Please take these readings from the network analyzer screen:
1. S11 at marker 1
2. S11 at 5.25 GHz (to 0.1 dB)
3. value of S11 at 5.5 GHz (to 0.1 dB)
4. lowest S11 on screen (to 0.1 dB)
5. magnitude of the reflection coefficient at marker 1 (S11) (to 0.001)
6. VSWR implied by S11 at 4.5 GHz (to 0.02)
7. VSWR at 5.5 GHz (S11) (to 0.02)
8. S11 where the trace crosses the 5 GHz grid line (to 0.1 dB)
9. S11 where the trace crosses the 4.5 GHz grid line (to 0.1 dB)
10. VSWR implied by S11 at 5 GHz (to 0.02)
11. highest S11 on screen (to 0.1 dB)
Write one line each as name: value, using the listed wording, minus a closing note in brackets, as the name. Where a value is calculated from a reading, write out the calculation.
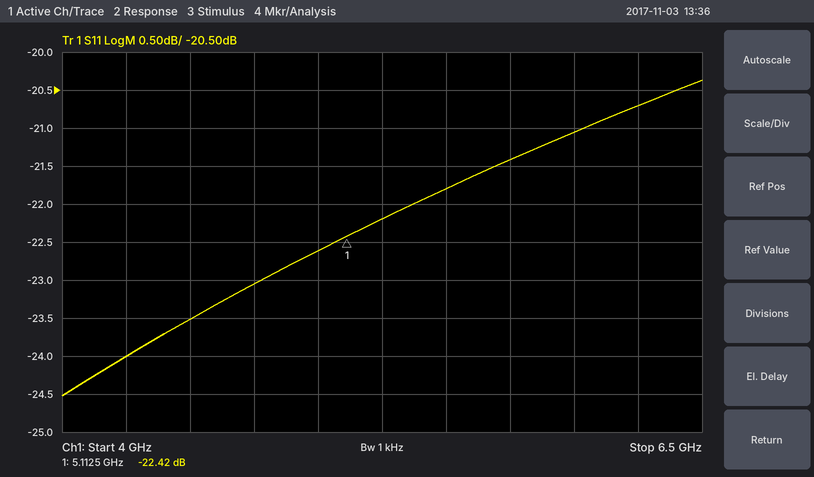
S11 at marker 1: -22.42 dB
S11 at 5.25 GHz: -22.2 dB
value of S11 at 5.5 GHz: -21.8 dB
lowest S11 on screen: -24.5 dB
magnitude of the reflection coefficient at marker 1 (S11): 10^(-22.42/20) ≈ 0.076
VSWR implied by S11 at 4.5 GHz: |Γ| = 10^(-23.5/20) = 0.0668; VSWR = (1 + 0.0668)/(1 − 0.0668) ≈ 1.14
VSWR at 5.5 GHz (S11): |Γ| = 10^(-21.8/20) = 0.0813; VSWR = (1 + 0.0813)/(1 − 0.0813) ≈ 1.18
S11 where the trace crosses the 5 GHz grid line: -22.6 dB
S11 where the trace crosses the 4.5 GHz grid line: -23.5 dB
VSWR implied by S11 at 5 GHz: |Γ| = 10^(-22.6/20) = 0.0741; VSWR = (1 + 0.0741)/(1 − 0.0741) ≈ 1.16
highest S11 on screen: -20.4 dB
